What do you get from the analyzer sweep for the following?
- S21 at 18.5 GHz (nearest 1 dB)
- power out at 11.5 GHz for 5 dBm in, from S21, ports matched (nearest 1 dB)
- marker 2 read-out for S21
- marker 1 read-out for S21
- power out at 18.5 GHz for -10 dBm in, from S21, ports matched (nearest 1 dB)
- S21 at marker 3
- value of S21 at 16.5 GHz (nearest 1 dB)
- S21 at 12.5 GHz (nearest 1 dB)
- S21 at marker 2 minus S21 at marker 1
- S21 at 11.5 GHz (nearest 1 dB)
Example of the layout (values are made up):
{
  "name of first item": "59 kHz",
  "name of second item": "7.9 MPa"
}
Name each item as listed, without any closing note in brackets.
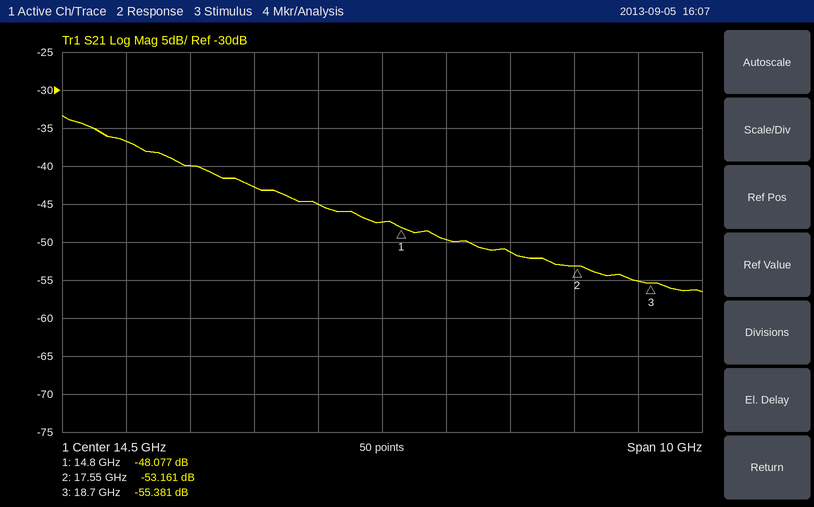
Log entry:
{
  "S21 at 18.5 GHz": "-55 dB",
  "power out at 11.5 GHz for 5 dBm in, from S21, ports matched": "-35 dBm",
  "marker 2 read-out for S21": "-53.161 dB",
  "marker 1 read-out for S21": "-48.077 dB",
  "power out at 18.5 GHz for -10 dBm in, from S21, ports matched": "-65 dBm",
  "S21 at marker 3": "-55.381 dB",
  "value of S21 at 16.5 GHz": "-51 dB",
  "S21 at 12.5 GHz": "-43 dB",
  "S21 at marker 2 minus S21 at marker 1": "-5.084 dB",
  "S21 at 11.5 GHz": "-40 dB"
}
